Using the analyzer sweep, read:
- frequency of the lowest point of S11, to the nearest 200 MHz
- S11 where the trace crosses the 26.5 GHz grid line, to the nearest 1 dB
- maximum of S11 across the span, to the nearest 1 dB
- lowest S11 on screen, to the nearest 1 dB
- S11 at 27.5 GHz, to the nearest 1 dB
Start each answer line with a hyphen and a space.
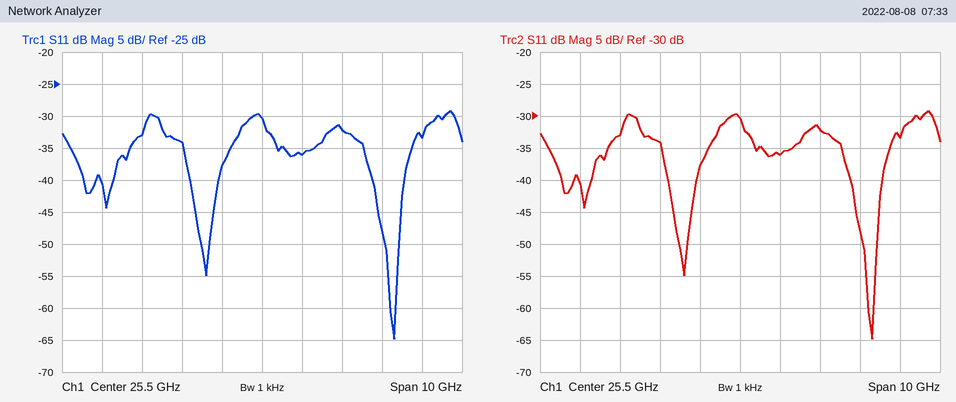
- 28.8 GHz
- -36 dB
- -29 dB
- -65 dB
- -32 dB
